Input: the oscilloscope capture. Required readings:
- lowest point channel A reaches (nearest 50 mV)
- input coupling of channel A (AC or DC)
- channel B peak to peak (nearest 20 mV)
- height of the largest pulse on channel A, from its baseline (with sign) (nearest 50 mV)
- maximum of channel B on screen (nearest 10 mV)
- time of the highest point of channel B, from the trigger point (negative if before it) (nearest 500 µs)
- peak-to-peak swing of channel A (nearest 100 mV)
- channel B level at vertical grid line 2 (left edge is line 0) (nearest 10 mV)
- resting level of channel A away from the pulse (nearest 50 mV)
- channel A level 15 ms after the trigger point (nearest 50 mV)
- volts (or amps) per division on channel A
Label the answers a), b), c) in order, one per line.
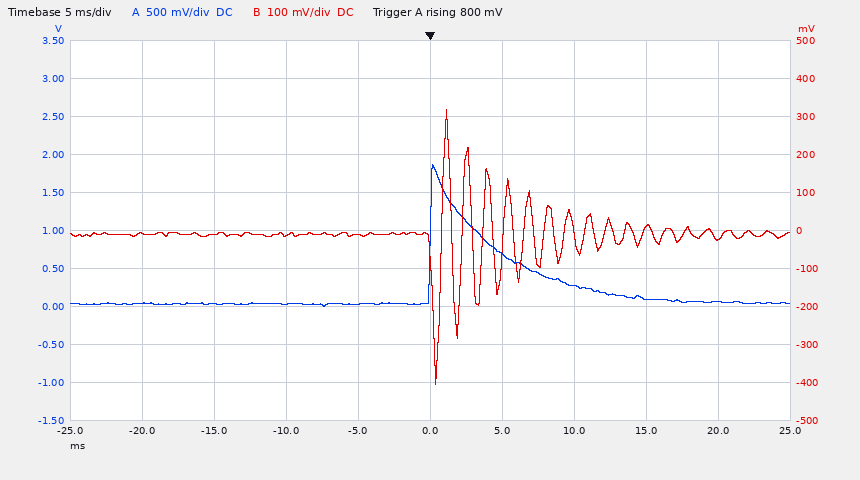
a) 0 mV
b) DC
c) 720 mV
d) +1.85 V
e) 320 mV
f) +1.0 ms
g) 1.90 V
h) -10 mV
i) 50 mV
j) 100 mV
k) 500 mV
